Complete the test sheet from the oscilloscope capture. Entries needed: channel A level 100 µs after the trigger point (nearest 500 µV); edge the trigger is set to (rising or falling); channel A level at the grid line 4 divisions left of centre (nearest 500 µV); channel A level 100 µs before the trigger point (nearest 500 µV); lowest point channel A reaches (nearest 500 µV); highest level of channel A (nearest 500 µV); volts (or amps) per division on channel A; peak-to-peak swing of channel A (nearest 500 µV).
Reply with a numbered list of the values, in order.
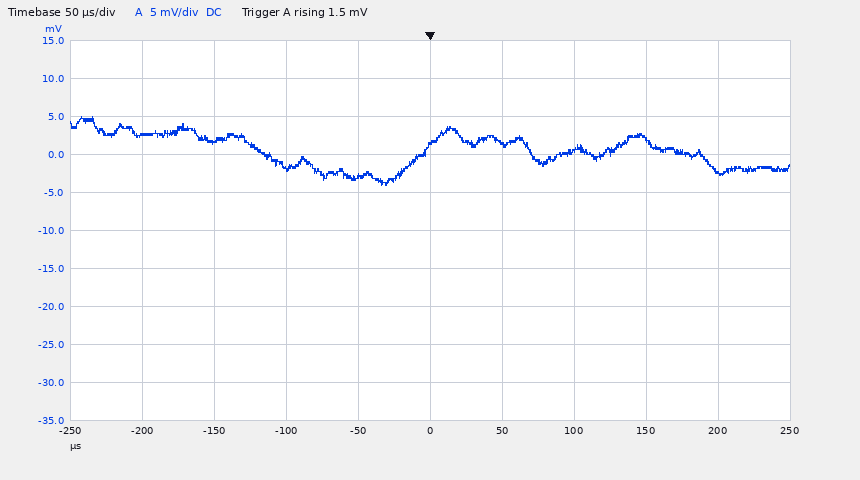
1. 500 µV
2. rising
3. 2.5 mV
4. -2.0 mV
5. -4.0 mV
6. 5.0 mV
7. 5 mV
8. 9.0 mV
